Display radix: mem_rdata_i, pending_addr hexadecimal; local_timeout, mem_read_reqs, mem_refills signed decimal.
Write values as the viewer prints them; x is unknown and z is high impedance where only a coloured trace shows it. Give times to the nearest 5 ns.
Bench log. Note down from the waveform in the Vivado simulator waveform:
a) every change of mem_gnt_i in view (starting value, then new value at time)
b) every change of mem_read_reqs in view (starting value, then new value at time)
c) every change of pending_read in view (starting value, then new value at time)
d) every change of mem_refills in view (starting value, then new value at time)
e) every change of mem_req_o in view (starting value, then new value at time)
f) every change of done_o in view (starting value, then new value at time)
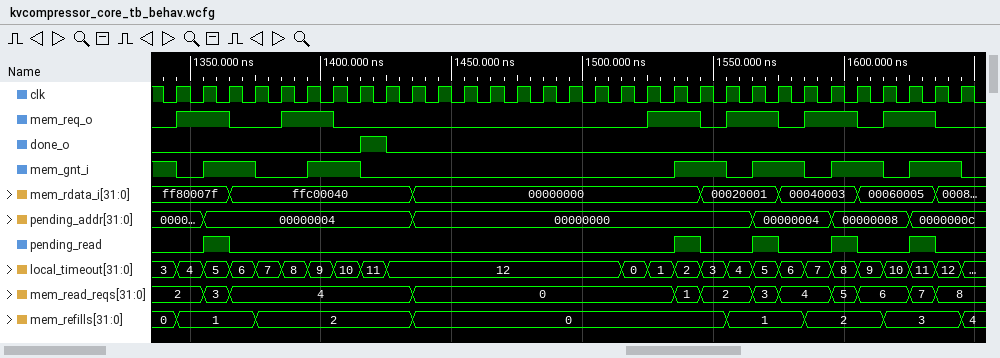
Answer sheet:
1, 0 at 1345 ns, 1 at 1355 ns, 0 at 1375 ns, 1 at 1395 ns, 0 at 1415 ns, 1 at 1535 ns, 0 at 1555 ns, 1 at 1565 ns, 0 at 1585 ns, 1 at 1595 ns, 0 at 1615 ns, 1 at 1625 ns, 0 at 1645 ns
2, 3 at 1355 ns, 4 at 1365 ns, 0 at 1435 ns, 1 at 1535 ns, 2 at 1545 ns, 3 at 1565 ns, 4 at 1575 ns, 5 at 1595 ns, 6 at 1605 ns, 7 at 1625 ns, 8 at 1635 ns
0, 1 at 1355 ns, 0 at 1365 ns, 1 at 1535 ns, 0 at 1545 ns, 1 at 1565 ns, 0 at 1575 ns, 1 at 1595 ns, 0 at 1605 ns, 1 at 1625 ns, 0 at 1635 ns
0, 1 at 1345 ns, 2 at 1375 ns, 0 at 1435 ns, 1 at 1555 ns, 2 at 1585 ns, 3 at 1615 ns, 4 at 1645 ns
0, 1 at 1345 ns, 0 at 1365 ns, 1 at 1385 ns, 0 at 1405 ns, 1 at 1525 ns, 0 at 1545 ns, 1 at 1555 ns, 0 at 1575 ns, 1 at 1585 ns, 0 at 1605 ns, 1 at 1615 ns, 0 at 1635 ns
0, 1 at 1415 ns, 0 at 1425 ns
